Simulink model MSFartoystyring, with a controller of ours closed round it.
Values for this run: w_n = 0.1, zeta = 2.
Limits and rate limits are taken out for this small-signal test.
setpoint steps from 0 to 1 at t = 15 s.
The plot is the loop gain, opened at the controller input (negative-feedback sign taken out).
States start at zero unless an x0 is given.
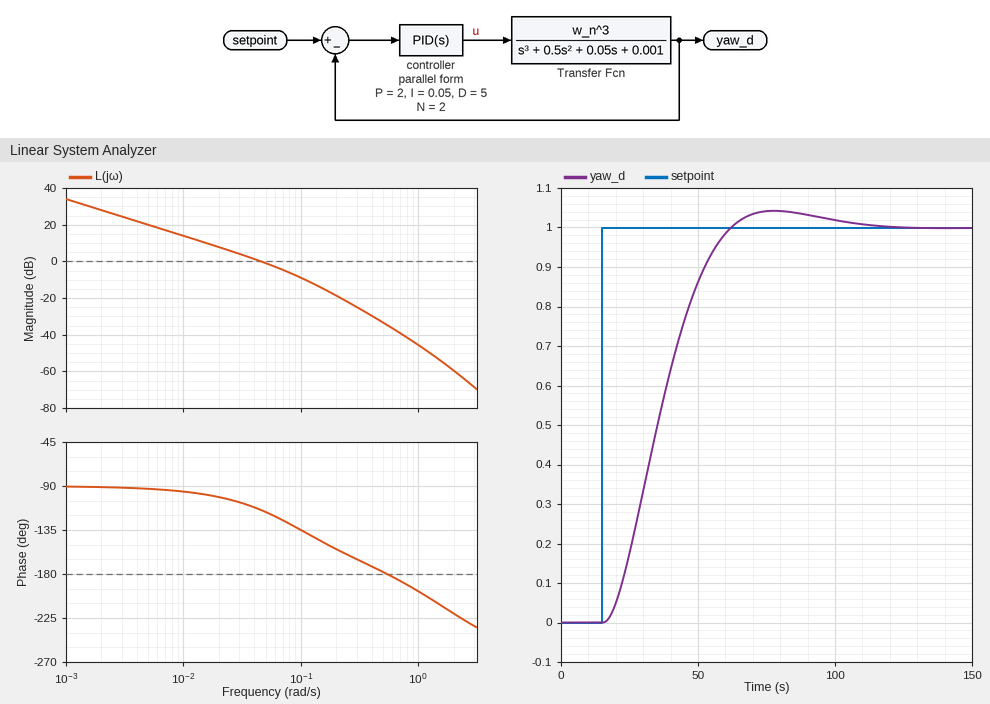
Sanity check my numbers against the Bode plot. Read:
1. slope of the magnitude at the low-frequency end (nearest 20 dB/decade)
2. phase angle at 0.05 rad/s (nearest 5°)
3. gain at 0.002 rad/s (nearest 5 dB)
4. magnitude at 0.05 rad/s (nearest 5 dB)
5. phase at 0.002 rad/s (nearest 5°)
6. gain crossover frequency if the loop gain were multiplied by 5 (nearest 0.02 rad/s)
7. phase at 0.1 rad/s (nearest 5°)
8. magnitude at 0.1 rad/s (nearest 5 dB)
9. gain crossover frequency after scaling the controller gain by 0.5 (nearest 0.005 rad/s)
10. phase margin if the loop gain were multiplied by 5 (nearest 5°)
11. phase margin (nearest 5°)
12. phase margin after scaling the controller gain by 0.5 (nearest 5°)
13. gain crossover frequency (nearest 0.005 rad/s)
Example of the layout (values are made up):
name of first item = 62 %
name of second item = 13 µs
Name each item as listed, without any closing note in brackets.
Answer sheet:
slope of the magnitude at the low-frequency end = -20 dB/decade
phase angle at 0.05 rad/s = -115°
gain at 0.002 rad/s = 30 dB
magnitude at 0.05 rad/s = 0 dB
phase at 0.002 rad/s = -90°
gain crossover frequency if the loop gain were multiplied by 5 = 0.14 rad/s
phase at 0.1 rad/s = -135°
magnitude at 0.1 rad/s = -10 dB
gain crossover frequency after scaling the controller gain by 0.5 = 0.025 rad/s
phase margin if the loop gain were multiplied by 5 = 35°
phase margin = 65°
phase margin after scaling the controller gain by 0.5 = 75°
gain crossover frequency = 0.045 rad/s
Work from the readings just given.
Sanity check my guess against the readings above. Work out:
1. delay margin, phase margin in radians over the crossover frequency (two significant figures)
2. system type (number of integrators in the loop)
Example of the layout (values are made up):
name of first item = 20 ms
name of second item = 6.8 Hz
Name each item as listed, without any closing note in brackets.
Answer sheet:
delay margin, phase margin in radians over the crossover frequency = 25 s
system type = 1
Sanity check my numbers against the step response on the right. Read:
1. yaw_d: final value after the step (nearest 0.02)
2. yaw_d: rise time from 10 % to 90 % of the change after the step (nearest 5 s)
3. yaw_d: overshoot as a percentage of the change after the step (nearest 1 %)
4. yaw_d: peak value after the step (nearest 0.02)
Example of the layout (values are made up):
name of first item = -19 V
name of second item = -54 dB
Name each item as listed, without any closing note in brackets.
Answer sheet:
yaw_d: final value after the step = 1.00
yaw_d: rise time from 10 % to 90 % of the change after the step = 30 s
yaw_d: overshoot as a percentage of the change after the step = 4 %
yaw_d: peak value after the step = 1.04
